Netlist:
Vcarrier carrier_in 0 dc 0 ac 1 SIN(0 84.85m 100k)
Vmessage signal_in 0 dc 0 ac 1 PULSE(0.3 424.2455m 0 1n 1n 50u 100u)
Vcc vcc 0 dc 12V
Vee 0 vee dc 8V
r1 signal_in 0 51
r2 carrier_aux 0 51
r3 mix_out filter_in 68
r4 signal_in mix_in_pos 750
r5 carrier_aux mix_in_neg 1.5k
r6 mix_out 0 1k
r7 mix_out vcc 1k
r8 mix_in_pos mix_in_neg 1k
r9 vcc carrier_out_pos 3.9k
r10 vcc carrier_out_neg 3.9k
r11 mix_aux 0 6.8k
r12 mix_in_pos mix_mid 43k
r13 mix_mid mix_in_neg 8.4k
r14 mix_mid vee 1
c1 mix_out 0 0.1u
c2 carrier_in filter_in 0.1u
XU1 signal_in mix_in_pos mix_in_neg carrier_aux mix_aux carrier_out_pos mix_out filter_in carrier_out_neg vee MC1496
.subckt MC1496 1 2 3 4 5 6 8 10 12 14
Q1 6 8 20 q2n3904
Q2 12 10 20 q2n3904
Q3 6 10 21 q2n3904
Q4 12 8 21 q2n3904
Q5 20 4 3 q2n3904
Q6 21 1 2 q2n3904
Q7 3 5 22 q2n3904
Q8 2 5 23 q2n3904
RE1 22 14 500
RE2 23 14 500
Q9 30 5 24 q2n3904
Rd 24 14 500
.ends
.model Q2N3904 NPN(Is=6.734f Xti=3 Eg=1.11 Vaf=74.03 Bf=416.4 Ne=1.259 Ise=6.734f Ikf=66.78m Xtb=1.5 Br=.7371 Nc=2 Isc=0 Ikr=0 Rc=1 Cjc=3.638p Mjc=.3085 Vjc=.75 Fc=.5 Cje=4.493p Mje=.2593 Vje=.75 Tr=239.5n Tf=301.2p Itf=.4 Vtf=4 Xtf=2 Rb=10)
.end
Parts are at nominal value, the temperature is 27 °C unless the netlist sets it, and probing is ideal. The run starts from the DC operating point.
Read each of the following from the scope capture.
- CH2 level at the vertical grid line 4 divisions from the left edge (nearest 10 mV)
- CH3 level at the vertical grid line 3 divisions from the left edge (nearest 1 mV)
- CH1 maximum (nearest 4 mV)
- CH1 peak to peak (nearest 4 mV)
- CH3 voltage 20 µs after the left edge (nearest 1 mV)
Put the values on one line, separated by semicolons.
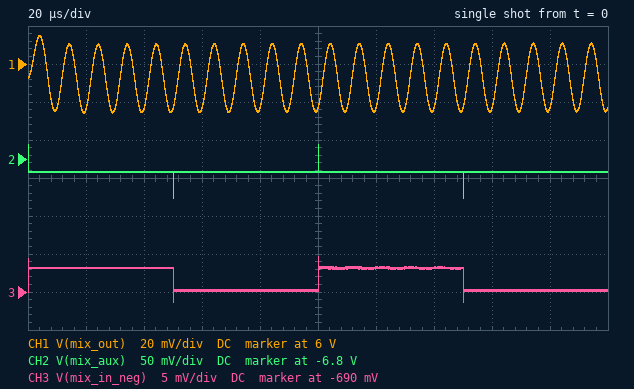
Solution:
-6.82 V; -690 mV; 6.016 V; 40 mV; -687 mV
